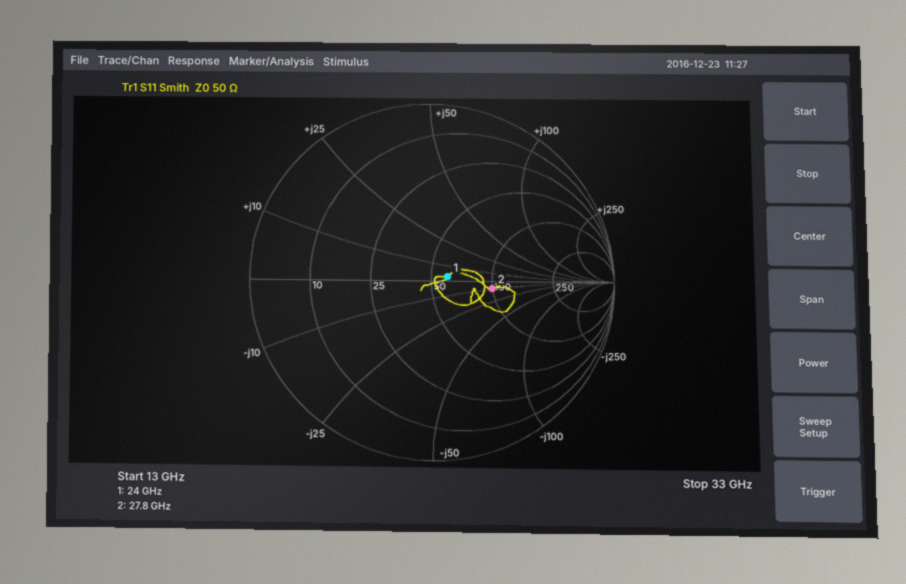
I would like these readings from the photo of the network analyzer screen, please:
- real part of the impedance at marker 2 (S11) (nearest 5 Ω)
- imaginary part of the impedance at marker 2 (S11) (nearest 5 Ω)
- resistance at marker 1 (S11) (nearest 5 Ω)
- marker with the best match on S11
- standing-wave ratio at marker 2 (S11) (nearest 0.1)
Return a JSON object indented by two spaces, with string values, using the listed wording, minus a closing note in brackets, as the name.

{
  "real part of the impedance at marker 2 (S11)": "100 Ω",
  "imaginary part of the impedance at marker 2 (S11)": "-10 Ω",
  "resistance at marker 1 (S11)": "60 Ω",
  "marker with the best match on S11": "marker 1",
  "standing-wave ratio at marker 2 (S11)": "2.0"
}
